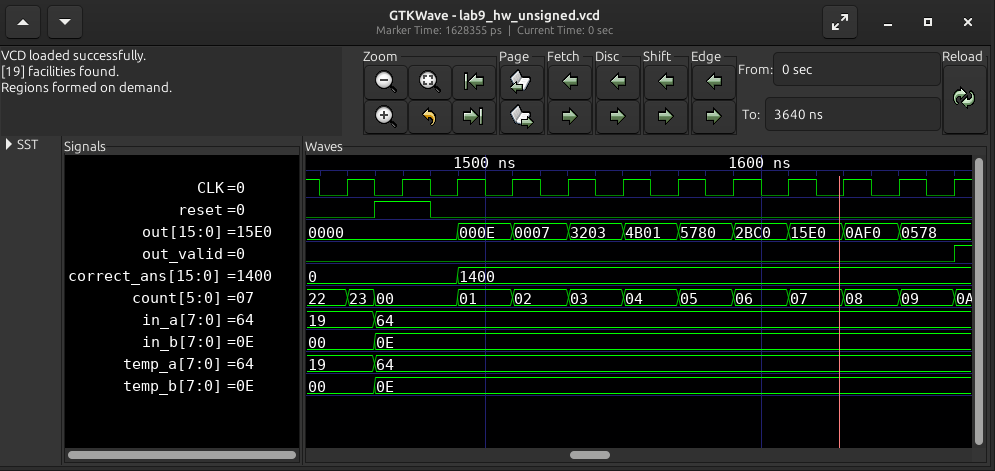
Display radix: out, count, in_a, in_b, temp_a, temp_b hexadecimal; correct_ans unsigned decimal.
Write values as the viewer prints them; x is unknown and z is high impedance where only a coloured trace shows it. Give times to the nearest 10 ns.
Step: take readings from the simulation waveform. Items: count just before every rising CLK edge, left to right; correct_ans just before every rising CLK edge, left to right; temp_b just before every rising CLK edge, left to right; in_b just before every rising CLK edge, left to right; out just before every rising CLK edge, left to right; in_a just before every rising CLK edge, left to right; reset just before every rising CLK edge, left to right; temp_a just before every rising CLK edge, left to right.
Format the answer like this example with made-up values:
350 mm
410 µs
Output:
22, 00, 00, 01, 02, 03, 04, 05, 06, 07, 08, 09
0, 0, 0, 1400, 1400, 1400, 1400, 1400, 1400, 1400, 1400, 1400
00, 0E, 0E, 0E, 0E, 0E, 0E, 0E, 0E, 0E, 0E, 0E
00, 0E, 0E, 0E, 0E, 0E, 0E, 0E, 0E, 0E, 0E, 0E
0000, 0000, 0000, 000E, 0007, 3203, 4B01, 5780, 2BC0, 15E0, 0AF0, 0578
19, 64, 64, 64, 64, 64, 64, 64, 64, 64, 64, 64
0 1 0 0 0 0 0 0 0 0 0 0
19, 64, 64, 64, 64, 64, 64, 64, 64, 64, 64, 64
